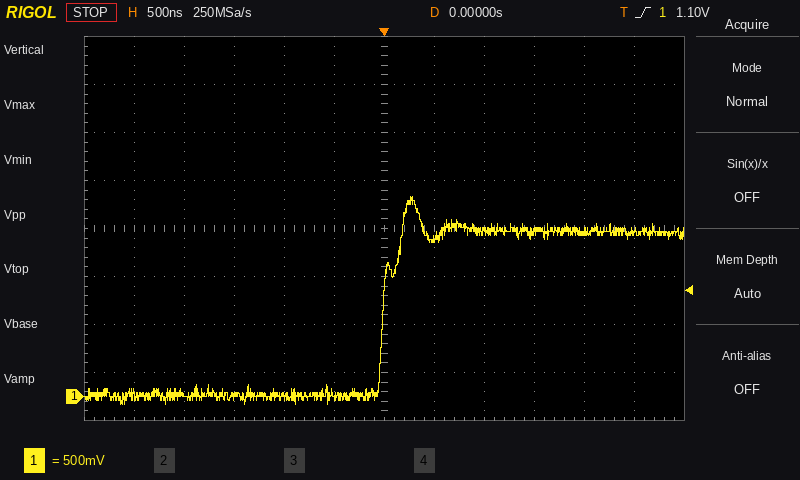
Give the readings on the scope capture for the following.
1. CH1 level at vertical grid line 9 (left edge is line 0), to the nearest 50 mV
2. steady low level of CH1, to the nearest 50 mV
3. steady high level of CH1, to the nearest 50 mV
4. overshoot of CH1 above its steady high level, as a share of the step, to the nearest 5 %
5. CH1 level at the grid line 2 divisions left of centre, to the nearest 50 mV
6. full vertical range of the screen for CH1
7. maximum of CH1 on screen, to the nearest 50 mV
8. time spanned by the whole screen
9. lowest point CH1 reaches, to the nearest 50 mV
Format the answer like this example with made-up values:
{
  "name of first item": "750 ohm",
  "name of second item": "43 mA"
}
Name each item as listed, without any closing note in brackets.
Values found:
{
  "CH1 level at vertical grid line 9 (left edge is line 0), to the nearest 50 mV": "1.70 V",
  "steady low level of CH1, to the nearest 50 mV": "0 mV",
  "steady high level of CH1, to the nearest 50 mV": "1.70 V",
  "overshoot of CH1 above its steady high level, as a share of the step, to the nearest 5 %": "20 %",
  "CH1 level at the grid line 2 divisions left of centre, to the nearest 50 mV": "0 mV",
  "full vertical range of the screen for CH1": "4 V",
  "maximum of CH1 on screen, to the nearest 50 mV": "2.10 V",
  "time spanned by the whole screen": "6 µs",
  "lowest point CH1 reaches, to the nearest 50 mV": "-100 mV"
}
